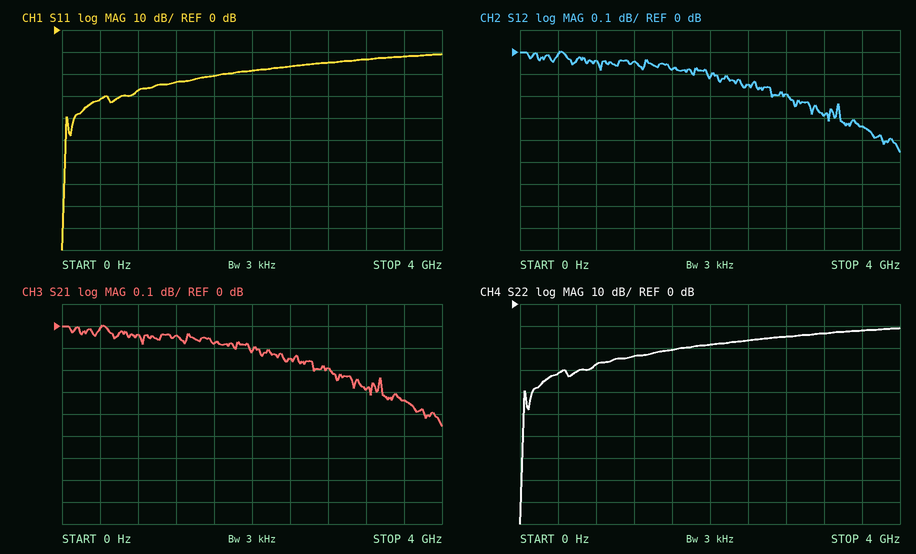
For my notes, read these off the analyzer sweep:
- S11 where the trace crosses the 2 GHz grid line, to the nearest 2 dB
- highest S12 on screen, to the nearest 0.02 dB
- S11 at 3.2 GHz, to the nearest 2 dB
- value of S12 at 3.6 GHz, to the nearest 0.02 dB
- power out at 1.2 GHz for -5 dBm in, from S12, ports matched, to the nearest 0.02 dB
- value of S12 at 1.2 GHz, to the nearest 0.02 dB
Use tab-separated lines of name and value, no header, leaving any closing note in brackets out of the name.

S11 where the trace crosses the 2 GHz grid line, to the nearest 2 dB	-18 dB
highest S12 on screen, to the nearest 0.02 dB	0.00 dB
S11 at 3.2 GHz, to the nearest 2 dB	-14 dB
value of S12 at 3.6 GHz, to the nearest 0.02 dB	-0.34 dB
power out at 1.2 GHz for -5 dBm in, from S12, ports matched, to the nearest 0.02 dB	-5.04 dBm
value of S12 at 1.2 GHz, to the nearest 0.02 dB	-0.04 dB
